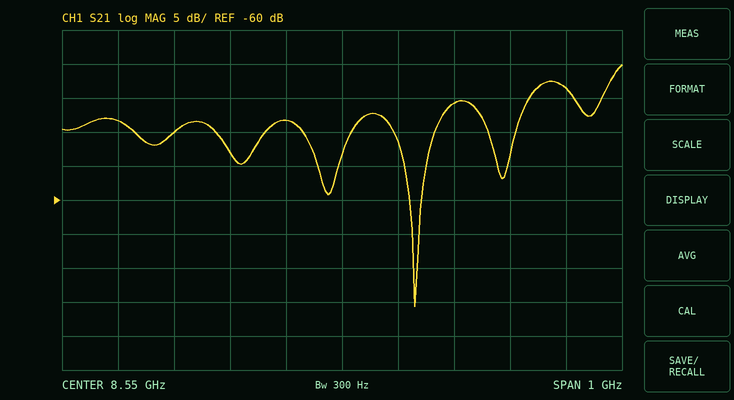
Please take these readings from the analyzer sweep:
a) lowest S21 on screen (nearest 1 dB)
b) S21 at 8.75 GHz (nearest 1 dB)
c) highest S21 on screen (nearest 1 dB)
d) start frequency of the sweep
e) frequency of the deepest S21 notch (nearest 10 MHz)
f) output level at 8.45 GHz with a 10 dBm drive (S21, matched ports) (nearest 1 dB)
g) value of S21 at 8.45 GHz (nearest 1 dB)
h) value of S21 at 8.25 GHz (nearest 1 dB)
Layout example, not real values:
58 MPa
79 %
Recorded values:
-76 dB
-46 dB
-40 dB
8.05 GHz
8.68 GHz
-38 dBm
-48 dB
-50 dB
